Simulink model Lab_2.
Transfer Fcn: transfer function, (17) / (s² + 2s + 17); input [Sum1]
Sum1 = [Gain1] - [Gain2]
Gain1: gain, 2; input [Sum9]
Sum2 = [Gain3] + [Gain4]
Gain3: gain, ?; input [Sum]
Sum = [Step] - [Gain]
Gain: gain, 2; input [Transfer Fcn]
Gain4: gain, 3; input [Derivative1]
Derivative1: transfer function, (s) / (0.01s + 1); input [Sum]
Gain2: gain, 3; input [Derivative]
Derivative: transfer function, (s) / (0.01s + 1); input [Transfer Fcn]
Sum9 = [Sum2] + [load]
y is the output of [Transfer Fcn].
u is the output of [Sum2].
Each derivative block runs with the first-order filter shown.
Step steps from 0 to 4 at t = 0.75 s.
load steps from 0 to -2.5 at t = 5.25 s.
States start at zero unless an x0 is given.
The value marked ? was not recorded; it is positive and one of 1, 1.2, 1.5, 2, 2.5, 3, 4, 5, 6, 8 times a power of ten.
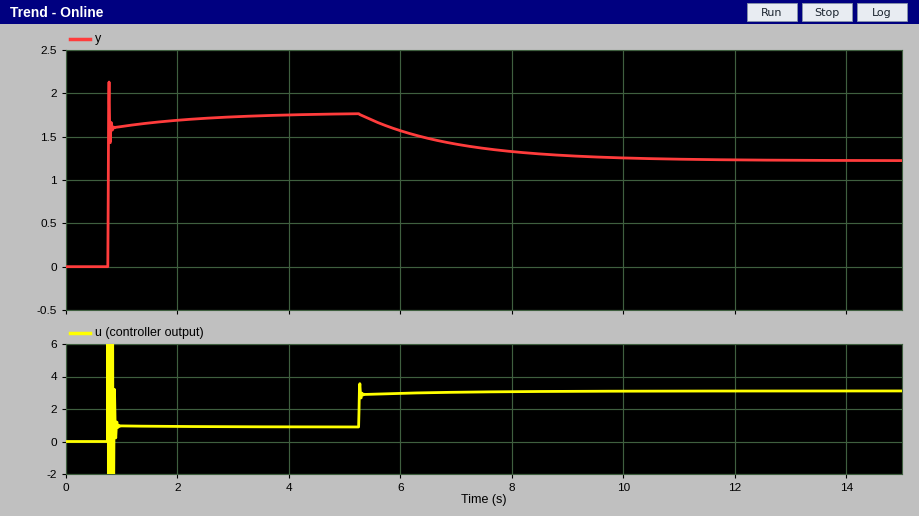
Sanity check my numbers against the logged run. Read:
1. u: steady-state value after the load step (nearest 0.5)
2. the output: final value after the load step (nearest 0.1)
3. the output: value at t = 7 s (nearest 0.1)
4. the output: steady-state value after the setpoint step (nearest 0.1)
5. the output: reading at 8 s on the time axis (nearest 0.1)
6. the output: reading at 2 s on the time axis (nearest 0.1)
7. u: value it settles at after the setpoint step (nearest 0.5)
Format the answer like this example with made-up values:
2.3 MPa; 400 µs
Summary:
3.0; 1.2; 1.4; 1.8; 1.3; 1.7; 1.0
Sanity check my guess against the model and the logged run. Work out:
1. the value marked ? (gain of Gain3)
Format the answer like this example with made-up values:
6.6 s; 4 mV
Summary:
2
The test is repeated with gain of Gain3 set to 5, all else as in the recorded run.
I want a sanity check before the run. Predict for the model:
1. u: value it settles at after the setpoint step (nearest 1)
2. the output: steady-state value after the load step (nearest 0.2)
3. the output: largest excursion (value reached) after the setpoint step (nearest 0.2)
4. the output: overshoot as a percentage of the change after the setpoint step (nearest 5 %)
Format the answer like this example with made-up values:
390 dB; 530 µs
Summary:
1; 1.6; 2.2; 15 %
